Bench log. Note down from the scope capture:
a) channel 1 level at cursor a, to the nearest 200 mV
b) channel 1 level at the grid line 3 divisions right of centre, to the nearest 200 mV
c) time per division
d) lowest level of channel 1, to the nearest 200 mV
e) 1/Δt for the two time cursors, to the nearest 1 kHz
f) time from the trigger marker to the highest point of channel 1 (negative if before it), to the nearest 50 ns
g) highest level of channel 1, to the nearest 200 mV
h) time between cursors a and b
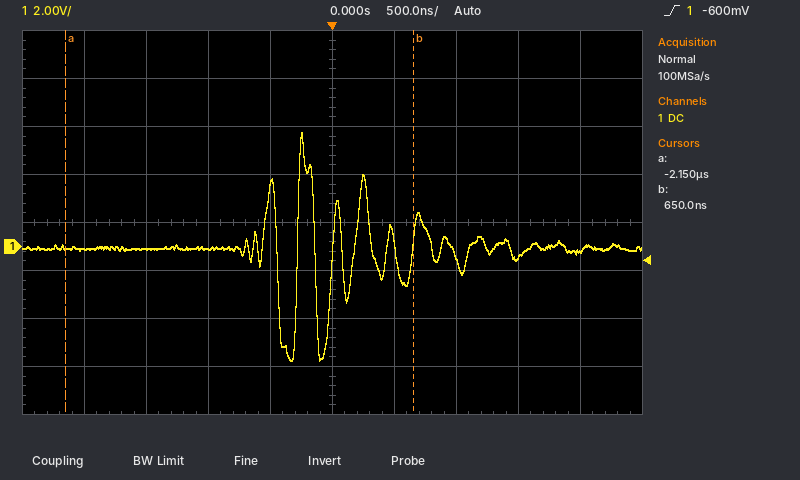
0.0 V
-400 mV
500 ns
-4.8 V
357 kHz
-250 ns
4.8 V
2.80 µs
